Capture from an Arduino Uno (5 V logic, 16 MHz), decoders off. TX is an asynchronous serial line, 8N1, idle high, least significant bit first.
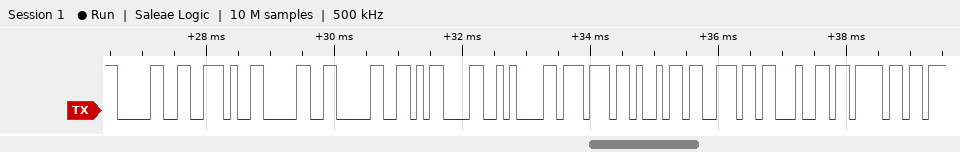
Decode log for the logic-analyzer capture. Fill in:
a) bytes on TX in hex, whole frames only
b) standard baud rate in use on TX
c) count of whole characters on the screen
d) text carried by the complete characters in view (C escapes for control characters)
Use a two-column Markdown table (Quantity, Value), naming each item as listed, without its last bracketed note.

| Quantity | Value |
|---|---|
| bytes on TX in hex, whole frames only | 30 2E 30 30 0D 0A 77 69 6E 64 6F |
| standard baud rate in use on TX | 9600 baud |
| count of whole characters on the screen | 11 |
| text carried by the complete characters in view | "0.00\r\nwindo" |
